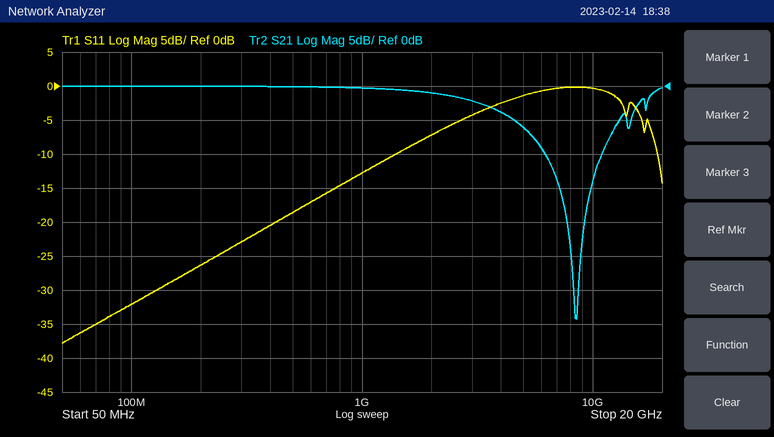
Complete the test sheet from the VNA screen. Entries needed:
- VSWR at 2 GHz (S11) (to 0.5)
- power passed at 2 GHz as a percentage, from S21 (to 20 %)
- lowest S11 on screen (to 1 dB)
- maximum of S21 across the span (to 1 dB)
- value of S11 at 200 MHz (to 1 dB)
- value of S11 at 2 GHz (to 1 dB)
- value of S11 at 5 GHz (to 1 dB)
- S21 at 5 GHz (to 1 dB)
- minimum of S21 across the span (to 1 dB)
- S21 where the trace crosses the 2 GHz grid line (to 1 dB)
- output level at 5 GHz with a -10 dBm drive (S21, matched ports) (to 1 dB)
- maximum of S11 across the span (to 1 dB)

2.5
80 %
-38 dB
0 dB
-26 dB
-7 dB
-1 dB
-6 dB
-34 dB
-1 dB
-16 dBm
0 dB
